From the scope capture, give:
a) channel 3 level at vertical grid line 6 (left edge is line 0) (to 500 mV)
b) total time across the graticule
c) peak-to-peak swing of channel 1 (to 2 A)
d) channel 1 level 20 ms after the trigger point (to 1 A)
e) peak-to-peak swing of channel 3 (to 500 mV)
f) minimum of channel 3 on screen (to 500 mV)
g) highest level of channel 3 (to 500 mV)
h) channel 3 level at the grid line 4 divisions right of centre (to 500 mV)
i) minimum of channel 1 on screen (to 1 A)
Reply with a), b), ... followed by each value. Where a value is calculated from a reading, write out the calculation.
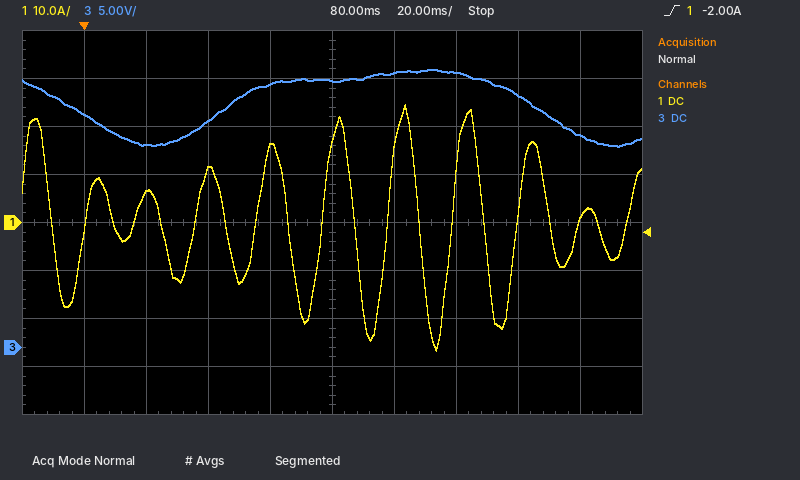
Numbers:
a) 28.5 V
b) 200 ms
c) 52 A
d) 6 A
e) 29.0 V − (21.0 V) = 8.0 V
f) 21.0 V
g) 29.0 V
h) 22.0 V
i) -27 A
